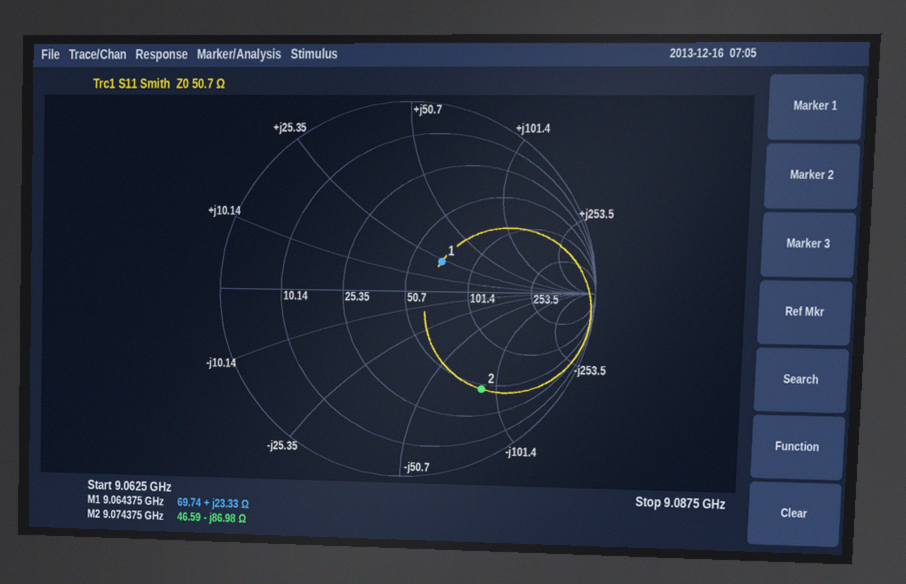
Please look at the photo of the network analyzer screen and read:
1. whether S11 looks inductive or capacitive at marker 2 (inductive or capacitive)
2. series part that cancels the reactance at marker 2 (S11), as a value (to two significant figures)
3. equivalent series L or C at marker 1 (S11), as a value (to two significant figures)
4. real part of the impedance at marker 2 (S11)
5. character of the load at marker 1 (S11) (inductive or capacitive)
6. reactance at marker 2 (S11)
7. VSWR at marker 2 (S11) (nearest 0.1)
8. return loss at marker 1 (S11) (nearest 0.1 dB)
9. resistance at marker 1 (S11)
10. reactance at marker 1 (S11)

capacitive
1.5 nH
410 pH
46.59 Ω
inductive
-86.98 Ω
5.0
12.2 dB
69.74 Ω
+23.33 Ω
